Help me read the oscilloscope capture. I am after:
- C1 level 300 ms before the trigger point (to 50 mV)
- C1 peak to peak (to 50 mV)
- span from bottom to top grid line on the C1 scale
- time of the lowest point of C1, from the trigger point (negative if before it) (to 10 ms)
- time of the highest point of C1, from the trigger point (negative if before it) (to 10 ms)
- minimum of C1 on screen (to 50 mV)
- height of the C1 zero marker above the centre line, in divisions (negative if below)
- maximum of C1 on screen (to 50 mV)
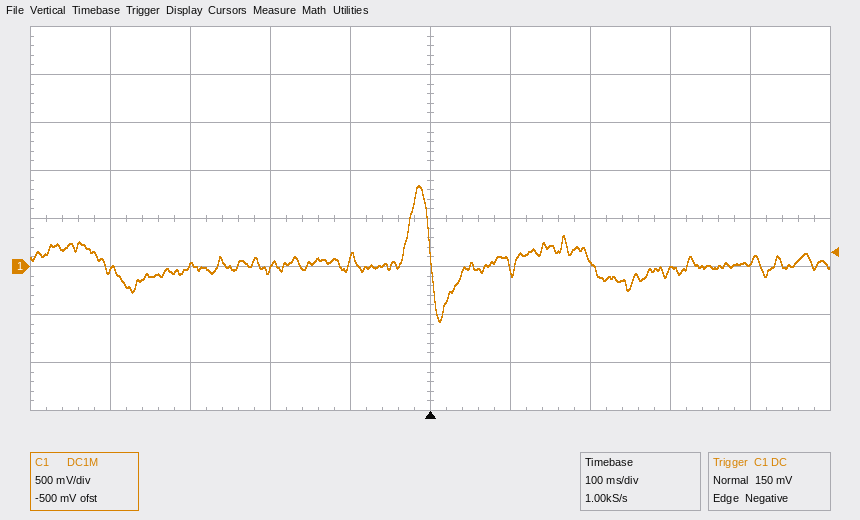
0 mV
1.40 V
4 V
+10 ms
-10 ms
-550 mV
-1.0 div
850 mV
